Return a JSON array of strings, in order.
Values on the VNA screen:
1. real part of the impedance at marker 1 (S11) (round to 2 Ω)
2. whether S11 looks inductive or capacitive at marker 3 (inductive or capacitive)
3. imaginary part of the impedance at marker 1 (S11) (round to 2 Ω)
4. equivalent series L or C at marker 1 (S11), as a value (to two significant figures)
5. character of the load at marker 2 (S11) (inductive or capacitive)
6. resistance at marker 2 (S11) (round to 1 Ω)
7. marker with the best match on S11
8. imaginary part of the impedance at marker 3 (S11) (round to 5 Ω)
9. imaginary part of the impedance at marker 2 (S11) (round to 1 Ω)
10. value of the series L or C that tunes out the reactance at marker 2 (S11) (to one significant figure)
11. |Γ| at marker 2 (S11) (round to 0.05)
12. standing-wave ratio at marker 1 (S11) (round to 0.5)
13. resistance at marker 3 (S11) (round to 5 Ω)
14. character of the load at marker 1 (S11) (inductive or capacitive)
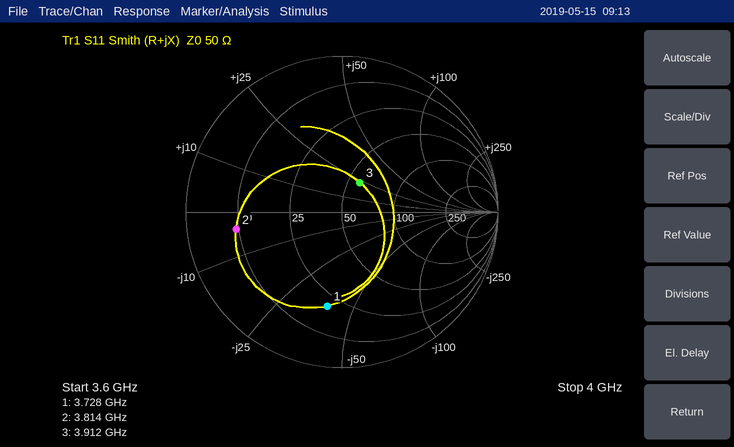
["20 Ω", "inductive", "-38 Ω", "1.1 pF", "capacitive", "9 Ω", "marker 3", "+25 Ω", "-4 Ω", "200 pH", "0.70", "4.0", "60 Ω", "capacitive"]
